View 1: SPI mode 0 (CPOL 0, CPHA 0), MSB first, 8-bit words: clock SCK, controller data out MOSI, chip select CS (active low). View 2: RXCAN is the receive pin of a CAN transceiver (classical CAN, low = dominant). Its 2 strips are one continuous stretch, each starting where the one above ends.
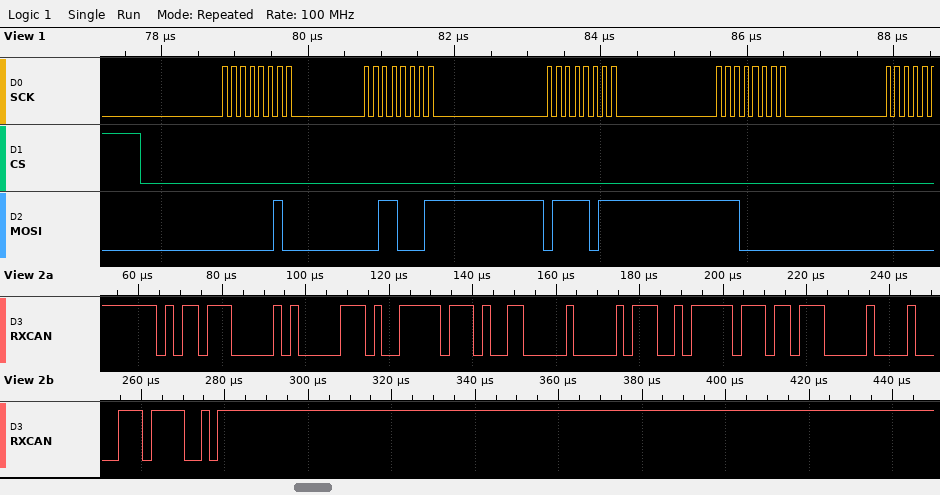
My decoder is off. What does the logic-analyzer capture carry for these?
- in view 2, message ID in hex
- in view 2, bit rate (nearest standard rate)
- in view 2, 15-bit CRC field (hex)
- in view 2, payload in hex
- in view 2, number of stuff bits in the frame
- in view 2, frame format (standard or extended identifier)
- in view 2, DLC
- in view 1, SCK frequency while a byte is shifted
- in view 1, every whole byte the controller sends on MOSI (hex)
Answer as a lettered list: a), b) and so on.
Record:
a) 0x5B8
b) 500 kbit/s
c) 0x43BC
d) 34 FF 4C 00 72 FF 6E 00
e) 7
f) standard
g) 8
h) 8 MHz
i) 02 31 7B E0
